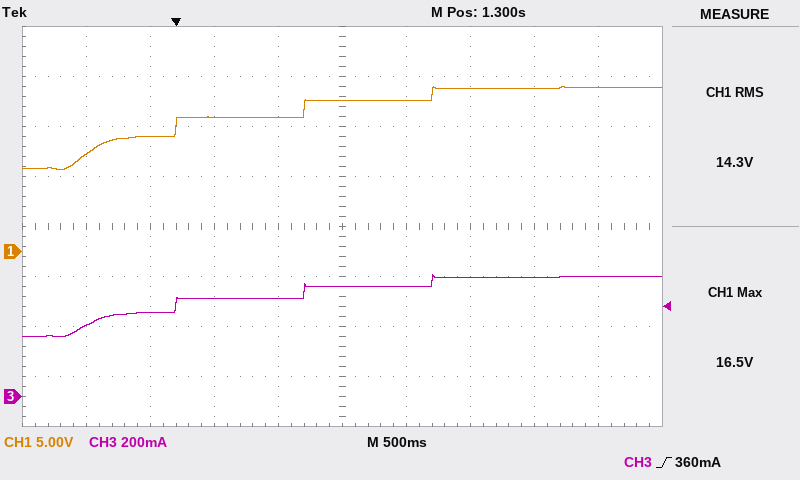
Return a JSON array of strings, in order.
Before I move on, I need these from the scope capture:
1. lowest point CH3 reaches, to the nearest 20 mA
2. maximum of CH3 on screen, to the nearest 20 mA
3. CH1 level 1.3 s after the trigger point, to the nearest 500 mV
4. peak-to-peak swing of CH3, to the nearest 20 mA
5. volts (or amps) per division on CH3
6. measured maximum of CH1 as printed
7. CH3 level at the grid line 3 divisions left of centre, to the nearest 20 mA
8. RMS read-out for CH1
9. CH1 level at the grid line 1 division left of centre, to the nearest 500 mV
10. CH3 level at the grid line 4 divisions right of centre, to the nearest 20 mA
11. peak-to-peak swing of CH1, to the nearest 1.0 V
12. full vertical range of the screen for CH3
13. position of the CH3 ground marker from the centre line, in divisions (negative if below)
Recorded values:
["240 mA", "480 mA", "15.0 V", "240 mA", "200 mA", "16.5 V", "340 mA", "14.3 V", "13.5 V", "480 mA", "8.0 V", "1.6 A", "-3.4 div"]
